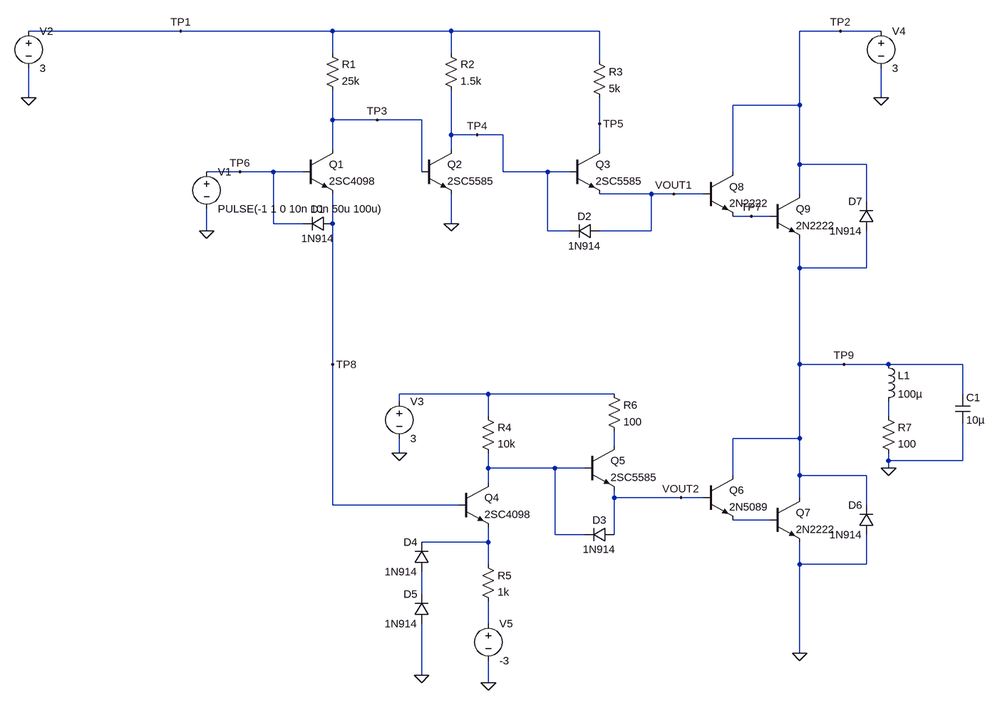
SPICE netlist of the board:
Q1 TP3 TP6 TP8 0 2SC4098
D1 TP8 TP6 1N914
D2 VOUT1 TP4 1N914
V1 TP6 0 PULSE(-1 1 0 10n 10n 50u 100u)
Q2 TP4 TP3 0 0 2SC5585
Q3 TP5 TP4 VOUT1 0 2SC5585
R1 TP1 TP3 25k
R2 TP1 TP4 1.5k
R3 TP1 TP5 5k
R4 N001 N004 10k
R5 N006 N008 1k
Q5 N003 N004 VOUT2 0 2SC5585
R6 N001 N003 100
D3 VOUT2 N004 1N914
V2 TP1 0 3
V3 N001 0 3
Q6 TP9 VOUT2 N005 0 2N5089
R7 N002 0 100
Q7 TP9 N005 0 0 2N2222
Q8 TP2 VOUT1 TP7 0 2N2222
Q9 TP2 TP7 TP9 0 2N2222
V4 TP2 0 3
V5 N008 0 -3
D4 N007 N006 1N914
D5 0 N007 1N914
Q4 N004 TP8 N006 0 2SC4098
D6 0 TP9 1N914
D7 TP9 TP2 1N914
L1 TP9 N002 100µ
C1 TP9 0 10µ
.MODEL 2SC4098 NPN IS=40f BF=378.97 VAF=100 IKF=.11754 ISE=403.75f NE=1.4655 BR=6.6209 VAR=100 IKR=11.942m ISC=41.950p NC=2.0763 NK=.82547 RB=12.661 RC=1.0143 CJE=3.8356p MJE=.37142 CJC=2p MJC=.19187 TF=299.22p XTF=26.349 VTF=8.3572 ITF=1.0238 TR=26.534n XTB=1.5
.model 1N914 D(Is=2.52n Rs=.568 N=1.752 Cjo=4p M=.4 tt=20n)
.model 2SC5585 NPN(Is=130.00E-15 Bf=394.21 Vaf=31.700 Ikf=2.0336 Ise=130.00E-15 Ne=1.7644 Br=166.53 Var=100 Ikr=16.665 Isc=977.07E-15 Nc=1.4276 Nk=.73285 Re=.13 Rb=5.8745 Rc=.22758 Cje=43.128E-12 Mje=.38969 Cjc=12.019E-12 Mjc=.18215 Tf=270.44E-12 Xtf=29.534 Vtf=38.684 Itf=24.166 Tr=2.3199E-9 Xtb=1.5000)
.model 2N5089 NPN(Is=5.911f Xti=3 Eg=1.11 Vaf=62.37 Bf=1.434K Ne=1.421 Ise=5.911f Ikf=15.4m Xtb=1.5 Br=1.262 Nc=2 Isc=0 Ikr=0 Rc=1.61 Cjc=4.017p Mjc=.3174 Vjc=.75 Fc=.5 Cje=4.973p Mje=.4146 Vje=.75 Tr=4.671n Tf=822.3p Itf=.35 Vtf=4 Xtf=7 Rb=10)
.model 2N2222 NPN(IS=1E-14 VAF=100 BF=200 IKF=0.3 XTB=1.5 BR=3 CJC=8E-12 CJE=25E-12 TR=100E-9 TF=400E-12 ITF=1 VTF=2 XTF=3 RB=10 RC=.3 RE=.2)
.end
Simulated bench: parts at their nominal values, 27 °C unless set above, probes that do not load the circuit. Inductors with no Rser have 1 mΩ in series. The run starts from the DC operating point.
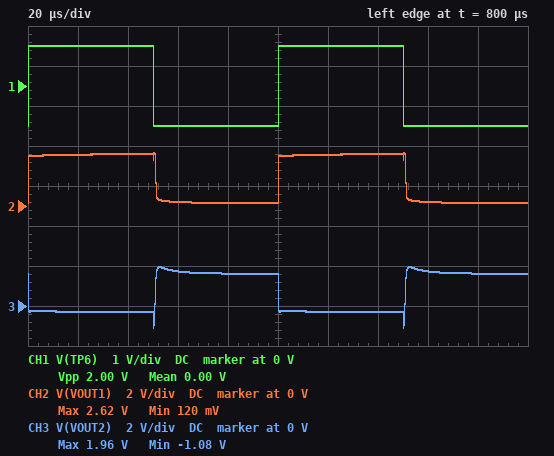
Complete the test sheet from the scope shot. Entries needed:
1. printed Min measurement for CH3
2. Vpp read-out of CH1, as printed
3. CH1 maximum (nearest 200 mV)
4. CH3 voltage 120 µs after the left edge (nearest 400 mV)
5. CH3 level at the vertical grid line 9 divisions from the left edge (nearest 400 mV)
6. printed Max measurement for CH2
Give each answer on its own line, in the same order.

-1.08 V
2.00 V
1.0 V
-400 mV
1.6 V
2.62 V
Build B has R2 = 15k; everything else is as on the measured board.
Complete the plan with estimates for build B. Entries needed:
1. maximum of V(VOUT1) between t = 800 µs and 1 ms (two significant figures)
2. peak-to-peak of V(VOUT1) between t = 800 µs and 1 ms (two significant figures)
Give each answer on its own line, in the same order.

2.7 V
2.6 V
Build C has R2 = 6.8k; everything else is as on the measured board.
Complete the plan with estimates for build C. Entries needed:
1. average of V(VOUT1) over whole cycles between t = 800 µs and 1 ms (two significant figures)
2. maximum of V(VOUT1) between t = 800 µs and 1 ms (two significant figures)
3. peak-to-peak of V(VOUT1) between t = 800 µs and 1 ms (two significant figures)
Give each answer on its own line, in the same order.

1.4 V
2.7 V
2.6 V
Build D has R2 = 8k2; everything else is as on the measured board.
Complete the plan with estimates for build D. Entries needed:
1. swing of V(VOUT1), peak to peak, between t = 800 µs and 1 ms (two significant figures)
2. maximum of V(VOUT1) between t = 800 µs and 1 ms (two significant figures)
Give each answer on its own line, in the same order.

2.6 V
2.7 V
